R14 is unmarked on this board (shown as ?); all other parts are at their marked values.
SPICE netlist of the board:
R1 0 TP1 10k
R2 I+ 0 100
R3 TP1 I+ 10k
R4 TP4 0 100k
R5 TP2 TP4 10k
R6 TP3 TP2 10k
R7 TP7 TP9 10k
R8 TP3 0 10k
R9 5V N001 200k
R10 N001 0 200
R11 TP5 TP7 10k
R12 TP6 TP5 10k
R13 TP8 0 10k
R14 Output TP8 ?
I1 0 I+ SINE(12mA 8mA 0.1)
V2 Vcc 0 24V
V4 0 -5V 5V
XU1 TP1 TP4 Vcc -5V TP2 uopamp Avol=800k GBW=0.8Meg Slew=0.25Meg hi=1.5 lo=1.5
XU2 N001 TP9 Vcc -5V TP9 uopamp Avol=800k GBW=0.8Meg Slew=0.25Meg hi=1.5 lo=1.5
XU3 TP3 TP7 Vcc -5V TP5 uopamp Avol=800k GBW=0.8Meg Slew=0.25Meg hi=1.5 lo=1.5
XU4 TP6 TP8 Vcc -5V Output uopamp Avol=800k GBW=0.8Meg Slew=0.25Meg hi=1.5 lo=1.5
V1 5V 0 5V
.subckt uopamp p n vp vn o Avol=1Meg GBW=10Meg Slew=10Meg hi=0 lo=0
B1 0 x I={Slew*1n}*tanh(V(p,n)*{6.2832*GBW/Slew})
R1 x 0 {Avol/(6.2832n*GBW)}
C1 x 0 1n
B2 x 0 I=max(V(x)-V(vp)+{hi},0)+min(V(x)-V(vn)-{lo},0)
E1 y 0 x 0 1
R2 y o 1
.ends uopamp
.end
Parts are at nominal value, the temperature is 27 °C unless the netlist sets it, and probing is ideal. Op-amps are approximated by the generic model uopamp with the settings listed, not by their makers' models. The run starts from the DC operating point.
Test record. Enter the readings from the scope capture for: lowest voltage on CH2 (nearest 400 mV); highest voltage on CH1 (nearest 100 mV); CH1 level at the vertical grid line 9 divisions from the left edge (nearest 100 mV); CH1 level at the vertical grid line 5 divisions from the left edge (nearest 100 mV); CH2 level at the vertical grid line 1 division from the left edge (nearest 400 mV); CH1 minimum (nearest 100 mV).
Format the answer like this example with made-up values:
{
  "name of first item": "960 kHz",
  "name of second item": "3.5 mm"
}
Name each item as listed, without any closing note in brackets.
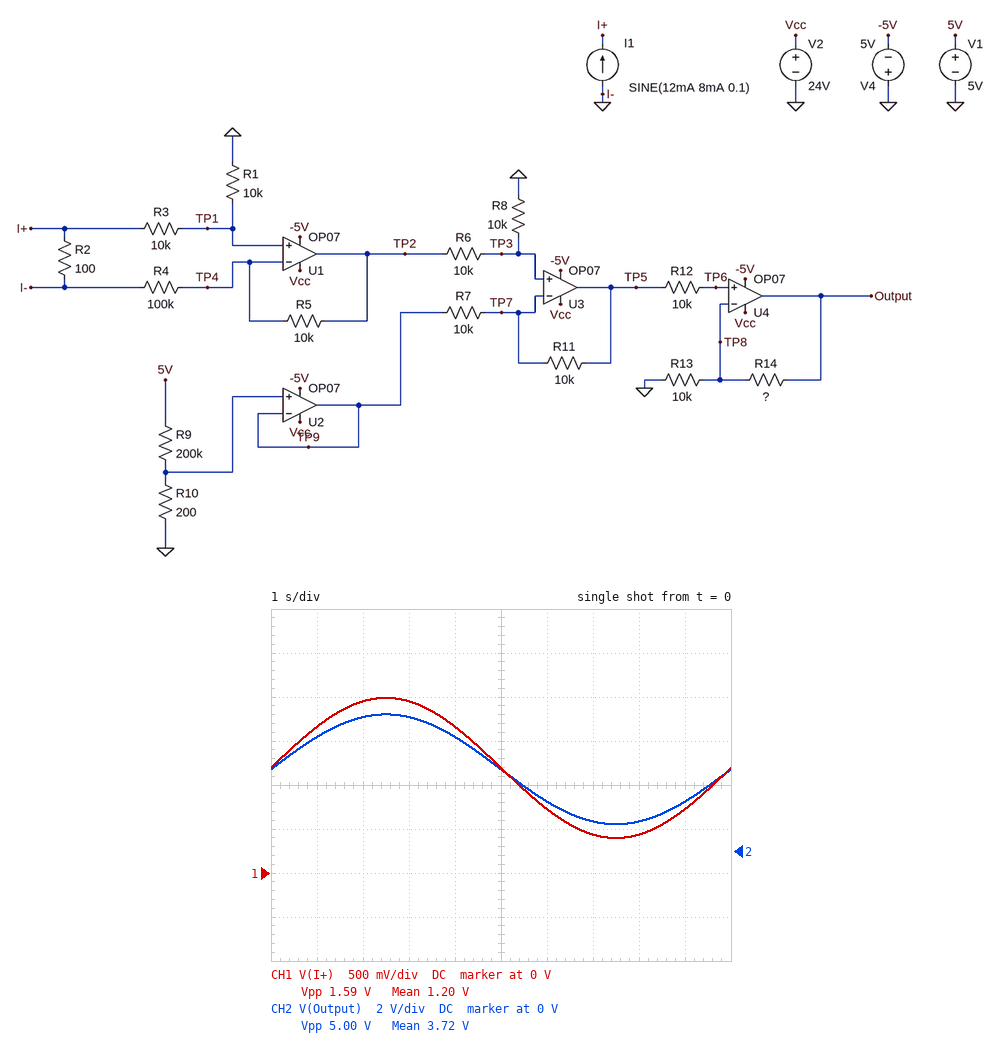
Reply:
{
  "lowest voltage on CH2": "1.2 V",
  "highest voltage on CH1": "2.0 V",
  "CH1 level at the vertical grid line 9 divisions from the left edge": "700 mV",
  "CH1 level at the vertical grid line 5 divisions from the left edge": "1.2 V",
  "CH2 level at the vertical grid line 1 division from the left edge": "5.2 V",
  "CH1 minimum": "400 mV"
}
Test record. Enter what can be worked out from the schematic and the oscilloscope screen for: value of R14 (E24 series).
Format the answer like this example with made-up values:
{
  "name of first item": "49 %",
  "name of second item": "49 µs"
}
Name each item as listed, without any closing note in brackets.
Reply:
{
  "value of R14": "47 kΩ"
}
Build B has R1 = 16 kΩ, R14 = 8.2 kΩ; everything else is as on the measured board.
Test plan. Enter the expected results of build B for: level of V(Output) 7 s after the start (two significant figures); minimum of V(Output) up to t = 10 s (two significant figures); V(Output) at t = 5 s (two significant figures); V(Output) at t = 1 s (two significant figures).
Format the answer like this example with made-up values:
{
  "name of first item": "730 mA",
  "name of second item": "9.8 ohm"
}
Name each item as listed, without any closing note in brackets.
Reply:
{
  "level of V(Output) 7 s after the start": "530 mV",
  "minimum of V(Output) up to t = 10 s": "480 mV",
  "V(Output) at t = 5 s": "1.5 V",
  "V(Output) at t = 1 s": "2.0 V"
}
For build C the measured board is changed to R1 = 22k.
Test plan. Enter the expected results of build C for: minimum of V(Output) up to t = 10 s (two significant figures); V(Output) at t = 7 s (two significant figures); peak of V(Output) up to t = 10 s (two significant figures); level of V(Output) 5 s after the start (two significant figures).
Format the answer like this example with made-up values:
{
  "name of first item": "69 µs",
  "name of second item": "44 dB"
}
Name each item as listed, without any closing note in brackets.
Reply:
{
  "minimum of V(Output) up to t = 10 s": "1.7 V",
  "V(Output) at t = 7 s": "1.9 V",
  "peak of V(Output) up to t = 10 s": "8.6 V",
  "level of V(Output) 5 s after the start": "5.1 V"
}
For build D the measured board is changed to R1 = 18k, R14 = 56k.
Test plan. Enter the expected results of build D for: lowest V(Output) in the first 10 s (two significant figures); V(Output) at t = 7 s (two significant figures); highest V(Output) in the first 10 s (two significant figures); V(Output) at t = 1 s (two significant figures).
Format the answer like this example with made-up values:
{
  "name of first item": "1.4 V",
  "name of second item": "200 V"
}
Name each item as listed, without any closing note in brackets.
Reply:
{
  "lowest V(Output) in the first 10 s": "1.8 V",
  "V(Output) at t = 7 s": "2.0 V",
  "highest V(Output) in the first 10 s": "9.3 V",
  "V(Output) at t = 1 s": "7.7 V"
}
